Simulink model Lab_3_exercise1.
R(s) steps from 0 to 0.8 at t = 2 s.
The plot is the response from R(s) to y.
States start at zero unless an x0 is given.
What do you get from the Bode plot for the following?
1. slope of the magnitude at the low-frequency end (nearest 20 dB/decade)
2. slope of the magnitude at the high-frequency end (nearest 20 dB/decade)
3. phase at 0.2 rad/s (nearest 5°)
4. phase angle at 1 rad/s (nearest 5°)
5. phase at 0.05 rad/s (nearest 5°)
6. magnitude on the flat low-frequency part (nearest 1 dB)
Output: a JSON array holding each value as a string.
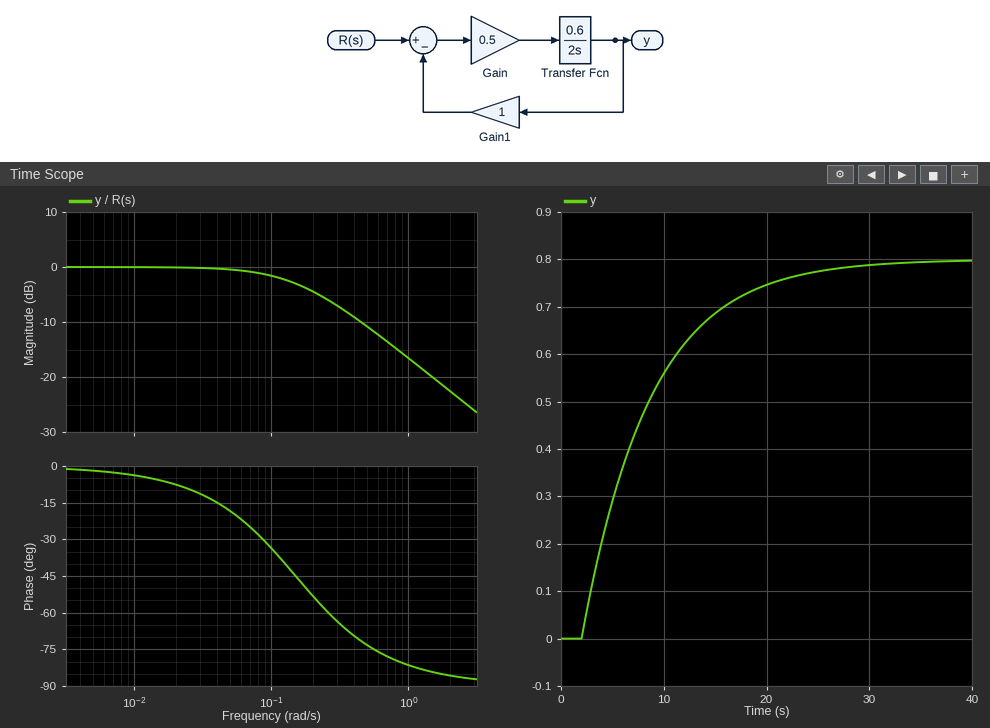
["0 dB/decade", "-20 dB/decade", "-55°", "-80°", "-20°", "0 dB"]
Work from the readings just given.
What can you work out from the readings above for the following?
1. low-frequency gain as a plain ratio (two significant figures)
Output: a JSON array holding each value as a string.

["1.0"]
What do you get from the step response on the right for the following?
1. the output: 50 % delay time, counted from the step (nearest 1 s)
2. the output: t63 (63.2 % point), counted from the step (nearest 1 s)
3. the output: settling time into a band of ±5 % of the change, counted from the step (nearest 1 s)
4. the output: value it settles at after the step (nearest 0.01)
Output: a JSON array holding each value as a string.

["5 s", "7 s", "20 s", "0.80"]
